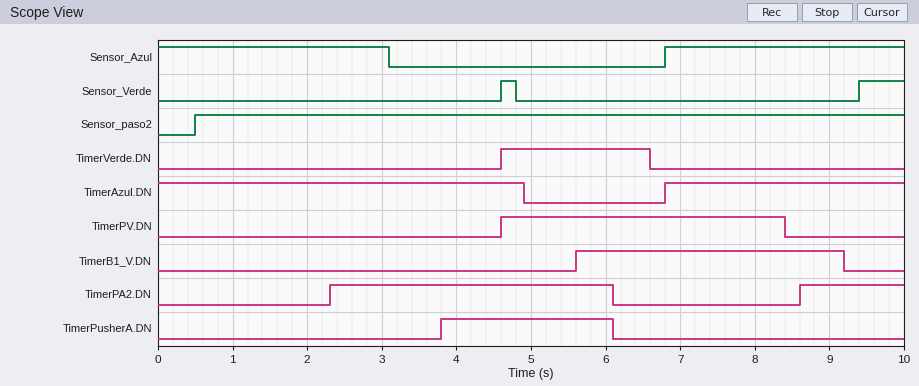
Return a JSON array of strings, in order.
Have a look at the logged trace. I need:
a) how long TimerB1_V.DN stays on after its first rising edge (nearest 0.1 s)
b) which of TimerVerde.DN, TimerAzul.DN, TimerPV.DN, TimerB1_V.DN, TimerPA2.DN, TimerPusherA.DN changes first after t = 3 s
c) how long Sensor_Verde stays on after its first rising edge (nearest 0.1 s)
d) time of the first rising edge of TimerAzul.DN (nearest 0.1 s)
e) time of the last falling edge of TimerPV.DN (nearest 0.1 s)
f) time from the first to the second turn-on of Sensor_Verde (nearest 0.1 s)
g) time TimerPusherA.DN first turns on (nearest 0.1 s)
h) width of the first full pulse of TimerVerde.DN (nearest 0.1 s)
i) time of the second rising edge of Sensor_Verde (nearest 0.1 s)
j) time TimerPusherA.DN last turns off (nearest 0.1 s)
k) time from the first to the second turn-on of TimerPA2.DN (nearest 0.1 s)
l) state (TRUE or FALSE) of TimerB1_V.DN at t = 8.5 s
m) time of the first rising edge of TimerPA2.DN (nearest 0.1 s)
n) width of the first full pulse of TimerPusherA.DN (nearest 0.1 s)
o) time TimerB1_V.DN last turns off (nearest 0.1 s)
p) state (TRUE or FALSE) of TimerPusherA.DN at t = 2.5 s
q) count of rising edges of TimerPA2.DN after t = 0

["3.6 s", "TimerPusherA.DN", "0.2 s", "6.8 s", "8.4 s", "4.8 s", "3.8 s", "2.0 s", "9.4 s", "6.1 s", "6.3 s", "TRUE", "2.3 s", "2.3 s", "9.2 s", "FALSE", "2"]
